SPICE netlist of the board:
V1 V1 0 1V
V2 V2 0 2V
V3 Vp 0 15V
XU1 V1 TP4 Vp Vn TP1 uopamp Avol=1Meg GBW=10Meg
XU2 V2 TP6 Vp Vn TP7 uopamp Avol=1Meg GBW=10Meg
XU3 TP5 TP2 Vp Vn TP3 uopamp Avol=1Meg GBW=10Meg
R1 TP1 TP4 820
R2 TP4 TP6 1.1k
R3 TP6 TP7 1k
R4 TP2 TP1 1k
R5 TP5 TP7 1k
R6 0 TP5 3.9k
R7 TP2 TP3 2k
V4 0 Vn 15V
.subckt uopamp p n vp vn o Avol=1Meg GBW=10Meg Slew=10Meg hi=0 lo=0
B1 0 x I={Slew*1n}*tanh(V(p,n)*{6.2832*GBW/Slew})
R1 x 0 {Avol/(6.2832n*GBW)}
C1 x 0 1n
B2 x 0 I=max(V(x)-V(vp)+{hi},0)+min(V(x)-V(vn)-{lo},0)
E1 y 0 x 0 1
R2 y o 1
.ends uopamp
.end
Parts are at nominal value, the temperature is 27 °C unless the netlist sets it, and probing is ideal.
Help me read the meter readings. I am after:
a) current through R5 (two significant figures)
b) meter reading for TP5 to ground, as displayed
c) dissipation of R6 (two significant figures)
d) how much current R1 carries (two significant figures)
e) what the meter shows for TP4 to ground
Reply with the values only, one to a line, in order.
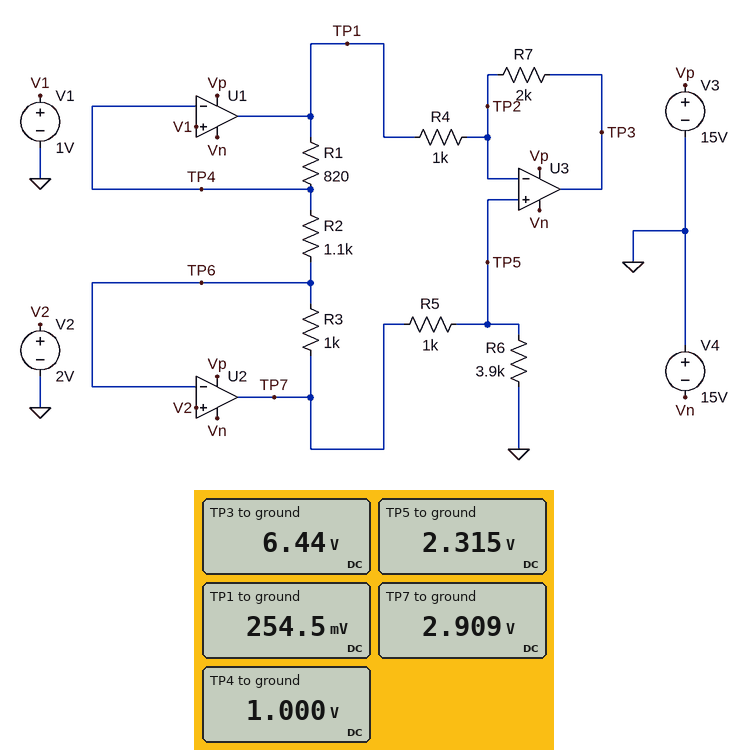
590 µA
2.315 V
1.4 mW
910 µA
1.000 V
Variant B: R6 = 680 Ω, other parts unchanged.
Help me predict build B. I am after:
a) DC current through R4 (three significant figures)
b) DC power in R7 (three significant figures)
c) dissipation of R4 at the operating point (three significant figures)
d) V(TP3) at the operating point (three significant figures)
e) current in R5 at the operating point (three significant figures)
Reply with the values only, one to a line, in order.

923 µA
1.70 mW
852 µW
3.02 V
1.73 mA
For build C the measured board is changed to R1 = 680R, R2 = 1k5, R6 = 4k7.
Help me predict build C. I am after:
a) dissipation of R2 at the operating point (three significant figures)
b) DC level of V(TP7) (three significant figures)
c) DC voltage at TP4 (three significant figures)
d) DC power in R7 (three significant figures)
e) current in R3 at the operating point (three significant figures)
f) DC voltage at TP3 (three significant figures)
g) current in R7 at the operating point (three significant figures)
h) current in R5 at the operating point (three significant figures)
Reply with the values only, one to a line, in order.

667 µW
2.67 V
1.00 V
5.46 mW
667 µA
5.50 V
1.65 mA
468 µA
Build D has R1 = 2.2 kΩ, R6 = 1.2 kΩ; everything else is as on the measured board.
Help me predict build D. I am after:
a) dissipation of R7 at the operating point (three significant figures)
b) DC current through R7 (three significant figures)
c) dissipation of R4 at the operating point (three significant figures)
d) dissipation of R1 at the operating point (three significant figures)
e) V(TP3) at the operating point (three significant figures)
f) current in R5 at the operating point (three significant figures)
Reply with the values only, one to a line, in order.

13.4 mW
2.59 mA
6.69 mW
1.82 mW
6.76 V
1.32 mA
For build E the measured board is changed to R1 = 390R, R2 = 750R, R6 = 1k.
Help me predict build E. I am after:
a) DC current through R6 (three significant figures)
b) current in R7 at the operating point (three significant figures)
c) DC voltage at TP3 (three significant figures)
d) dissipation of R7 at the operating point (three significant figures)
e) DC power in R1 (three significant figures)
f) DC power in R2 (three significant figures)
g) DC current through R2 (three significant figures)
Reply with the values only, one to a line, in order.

1.67 mA
1.19 mA
4.04 V
2.82 mW
693 µW
1.33 mW
1.33 mA
